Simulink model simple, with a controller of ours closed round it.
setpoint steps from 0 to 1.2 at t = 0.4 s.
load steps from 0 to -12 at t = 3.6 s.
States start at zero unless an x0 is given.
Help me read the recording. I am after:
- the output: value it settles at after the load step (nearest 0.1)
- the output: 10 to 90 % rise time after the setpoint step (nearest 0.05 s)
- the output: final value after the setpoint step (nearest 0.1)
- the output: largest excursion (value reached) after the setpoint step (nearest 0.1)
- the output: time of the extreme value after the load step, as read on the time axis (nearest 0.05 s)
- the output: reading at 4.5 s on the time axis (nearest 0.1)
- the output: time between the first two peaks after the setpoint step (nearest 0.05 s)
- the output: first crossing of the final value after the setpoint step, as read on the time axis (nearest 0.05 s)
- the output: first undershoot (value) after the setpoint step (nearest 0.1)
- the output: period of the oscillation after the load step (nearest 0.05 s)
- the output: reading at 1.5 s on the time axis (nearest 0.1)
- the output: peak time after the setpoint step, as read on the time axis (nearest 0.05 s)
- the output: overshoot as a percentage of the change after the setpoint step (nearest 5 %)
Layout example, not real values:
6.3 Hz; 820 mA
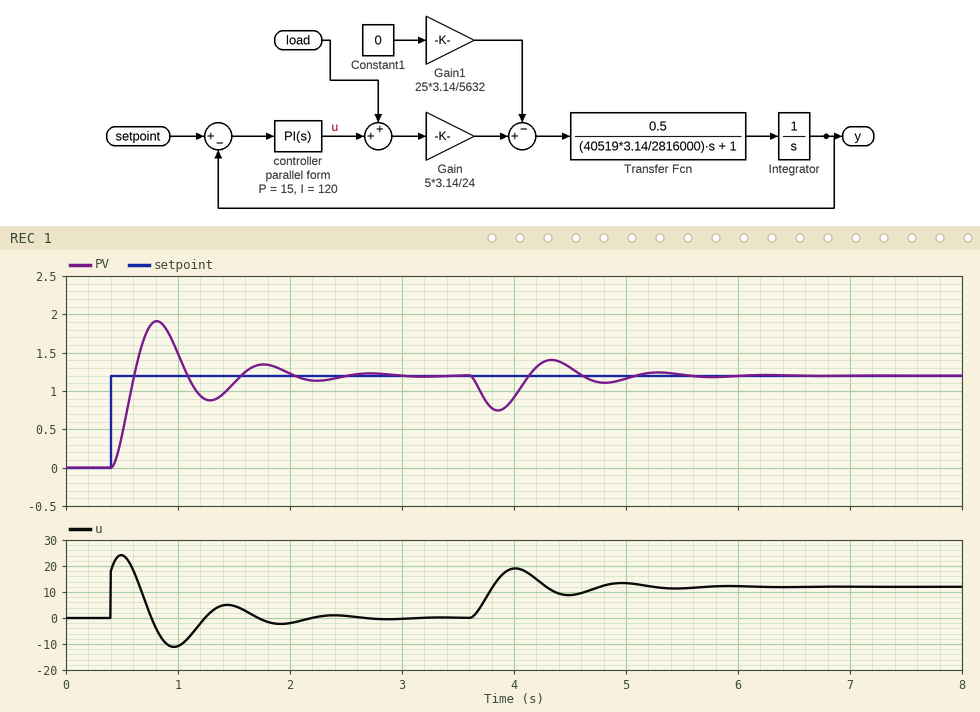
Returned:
1.2; 0.15 s; 1.2; 1.9; 3.85 s; 1.3; 0.95 s; 0.60 s; 0.9; 0.95 s; 1.1; 0.80 s; 60 %
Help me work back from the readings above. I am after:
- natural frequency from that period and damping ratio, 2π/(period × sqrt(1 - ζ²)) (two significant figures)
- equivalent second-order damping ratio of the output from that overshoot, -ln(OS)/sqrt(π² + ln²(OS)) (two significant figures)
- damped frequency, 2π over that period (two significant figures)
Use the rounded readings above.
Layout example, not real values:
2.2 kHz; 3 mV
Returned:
6.7 rad/s; 0.16; 6.6 rad/s
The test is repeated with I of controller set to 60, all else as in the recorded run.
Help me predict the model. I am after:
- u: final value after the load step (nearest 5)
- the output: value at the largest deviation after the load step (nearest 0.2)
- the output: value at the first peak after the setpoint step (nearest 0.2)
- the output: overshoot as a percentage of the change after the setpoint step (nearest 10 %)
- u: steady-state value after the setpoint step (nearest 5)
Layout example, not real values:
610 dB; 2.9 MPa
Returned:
10; 0.6; 1.6; 40 %; 0
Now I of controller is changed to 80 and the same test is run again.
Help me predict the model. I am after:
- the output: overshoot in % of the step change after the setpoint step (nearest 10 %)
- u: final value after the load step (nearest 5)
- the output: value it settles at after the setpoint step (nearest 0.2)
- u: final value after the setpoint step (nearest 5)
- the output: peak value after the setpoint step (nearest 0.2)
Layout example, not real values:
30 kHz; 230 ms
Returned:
50 %; 10; 1.2; 0; 1.8
